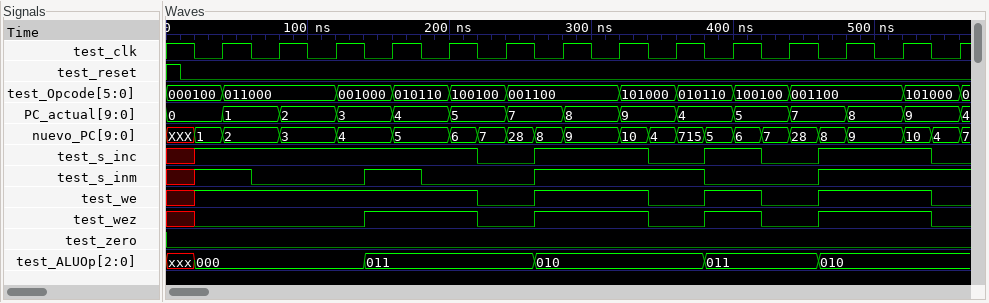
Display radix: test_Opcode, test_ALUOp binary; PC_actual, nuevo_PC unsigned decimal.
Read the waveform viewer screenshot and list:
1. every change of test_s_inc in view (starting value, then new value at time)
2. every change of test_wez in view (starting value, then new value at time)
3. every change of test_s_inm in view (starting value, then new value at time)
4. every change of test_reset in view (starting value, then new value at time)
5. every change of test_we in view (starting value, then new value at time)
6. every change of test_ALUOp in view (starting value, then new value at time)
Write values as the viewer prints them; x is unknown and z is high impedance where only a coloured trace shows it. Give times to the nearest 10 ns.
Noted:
x, 1 at 20 ns, 0 at 220 ns, 1 at 260 ns, 0 at 340 ns, 1 at 380 ns, 0 at 420 ns, 1 at 460 ns, 0 at 540 ns
x, 0 at 20 ns, 1 at 140 ns, 0 at 220 ns, 1 at 260 ns, 0 at 340 ns, 1 at 380 ns, 0 at 420 ns, 1 at 460 ns, 0 at 540 ns
x, 1 at 20 ns, 0 at 60 ns, 1 at 140 ns, 0 at 180 ns, 1 at 260 ns, 0 at 380 ns, 1 at 460 ns
1, 0 at 10 ns
x, 1 at 20 ns, 0 at 220 ns, 1 at 260 ns, 0 at 340 ns, 1 at 380 ns, 0 at 420 ns, 1 at 460 ns, 0 at 540 ns
xxx, 000 at 20 ns, 011 at 140 ns, 010 at 260 ns, 011 at 380 ns, 010 at 460 ns
